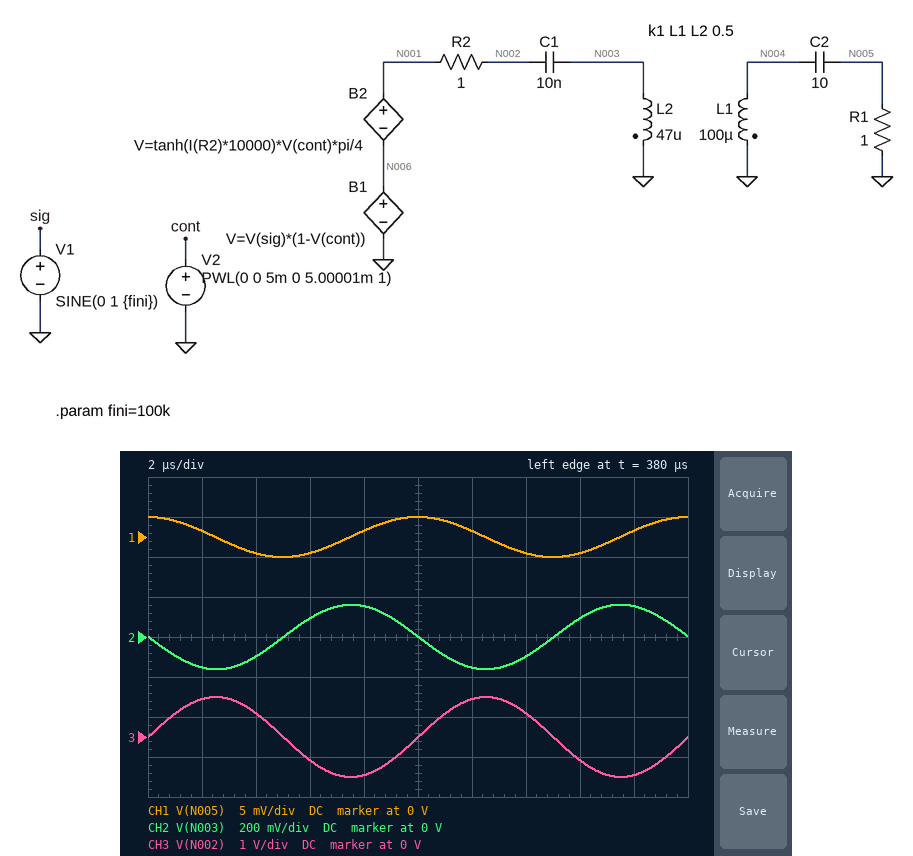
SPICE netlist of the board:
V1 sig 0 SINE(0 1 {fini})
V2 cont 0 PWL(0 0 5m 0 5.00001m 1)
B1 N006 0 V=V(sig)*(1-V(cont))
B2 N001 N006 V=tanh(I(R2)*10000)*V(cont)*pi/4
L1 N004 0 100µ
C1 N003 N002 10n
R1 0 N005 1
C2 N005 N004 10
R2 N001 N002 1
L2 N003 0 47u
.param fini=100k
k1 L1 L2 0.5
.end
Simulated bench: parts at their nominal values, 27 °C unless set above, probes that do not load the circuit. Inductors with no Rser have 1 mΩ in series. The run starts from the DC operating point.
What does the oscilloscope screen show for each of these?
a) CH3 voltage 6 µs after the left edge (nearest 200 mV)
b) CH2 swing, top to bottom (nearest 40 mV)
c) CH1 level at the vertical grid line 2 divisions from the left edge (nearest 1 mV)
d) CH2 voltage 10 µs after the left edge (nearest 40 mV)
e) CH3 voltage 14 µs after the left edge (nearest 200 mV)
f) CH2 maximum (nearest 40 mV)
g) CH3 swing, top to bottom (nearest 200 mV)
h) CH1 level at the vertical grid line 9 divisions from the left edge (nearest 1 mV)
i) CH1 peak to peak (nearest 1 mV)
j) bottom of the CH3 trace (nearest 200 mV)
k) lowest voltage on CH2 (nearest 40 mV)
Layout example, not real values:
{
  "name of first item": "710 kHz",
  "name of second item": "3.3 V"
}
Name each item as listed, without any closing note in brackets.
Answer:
{
  "CH3 voltage 6 µs after the left edge": "-600 mV",
  "CH2 swing, top to bottom": "320 mV",
  "CH1 level at the vertical grid line 2 divisions from the left edge": "-2 mV",
  "CH2 voltage 10 µs after the left edge": "0 V",
  "CH3 voltage 14 µs after the left edge": "600 mV",
  "CH2 maximum": "160 mV",
  "CH3 swing, top to bottom": "2.0 V",
  "CH1 level at the vertical grid line 9 divisions from the left edge": "1 mV",
  "CH1 peak to peak": "5 mV",
  "bottom of the CH3 trace": "-1.0 V",
  "lowest voltage on CH2": "-160 mV"
}
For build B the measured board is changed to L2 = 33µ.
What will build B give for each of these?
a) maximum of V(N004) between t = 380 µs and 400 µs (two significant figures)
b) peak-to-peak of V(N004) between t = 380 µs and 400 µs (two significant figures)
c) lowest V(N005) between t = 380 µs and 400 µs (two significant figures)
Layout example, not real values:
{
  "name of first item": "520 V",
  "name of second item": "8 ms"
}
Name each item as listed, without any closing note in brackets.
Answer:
{
  "maximum of V(N004) between t = 380 µs and 400 µs": "2.0 mV",
  "peak-to-peak of V(N004) between t = 380 µs and 400 µs": "4.0 mV",
  "lowest V(N005) between t = 380 µs and 400 µs": "-2.0 mV"
}
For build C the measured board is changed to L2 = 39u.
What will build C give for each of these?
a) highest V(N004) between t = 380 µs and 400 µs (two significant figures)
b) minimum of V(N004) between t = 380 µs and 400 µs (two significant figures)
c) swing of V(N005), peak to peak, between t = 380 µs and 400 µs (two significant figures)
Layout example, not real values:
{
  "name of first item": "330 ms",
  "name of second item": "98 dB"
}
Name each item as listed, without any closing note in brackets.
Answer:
{
  "highest V(N004) between t = 380 µs and 400 µs": "2.2 mV",
  "minimum of V(N004) between t = 380 µs and 400 µs": "-2.2 mV",
  "swing of V(N005), peak to peak, between t = 380 µs and 400 µs": "4.4 mV"
}
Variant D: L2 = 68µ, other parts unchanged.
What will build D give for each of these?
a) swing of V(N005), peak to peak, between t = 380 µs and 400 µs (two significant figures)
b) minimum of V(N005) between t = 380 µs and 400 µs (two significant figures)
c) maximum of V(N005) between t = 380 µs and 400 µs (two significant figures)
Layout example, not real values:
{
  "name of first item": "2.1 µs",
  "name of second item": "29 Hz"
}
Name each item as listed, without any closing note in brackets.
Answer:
{
  "swing of V(N005), peak to peak, between t = 380 µs and 400 µs": "6.5 mV",
  "minimum of V(N005) between t = 380 µs and 400 µs": "-3.3 mV",
  "maximum of V(N005) between t = 380 µs and 400 µs": "3.3 mV"
}
